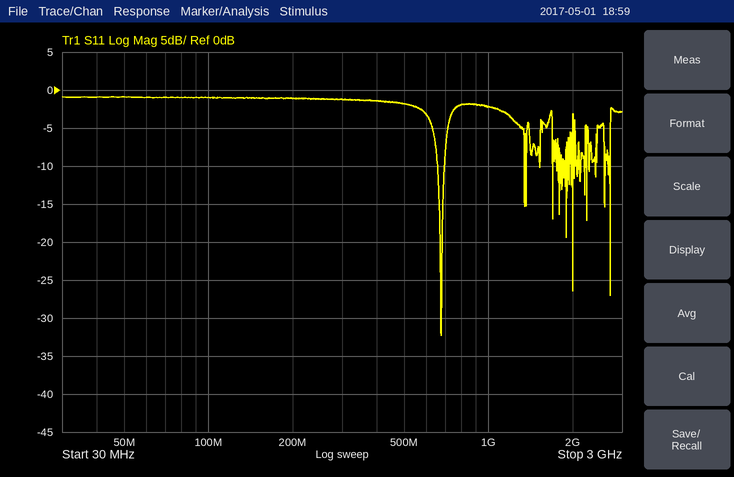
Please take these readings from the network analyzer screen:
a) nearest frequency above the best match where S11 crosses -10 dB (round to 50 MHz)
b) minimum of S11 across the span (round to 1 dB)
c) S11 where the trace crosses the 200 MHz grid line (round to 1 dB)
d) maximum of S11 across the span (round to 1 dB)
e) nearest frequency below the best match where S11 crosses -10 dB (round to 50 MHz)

700 MHz
-32 dB
-1 dB
-1 dB
650 MHz
